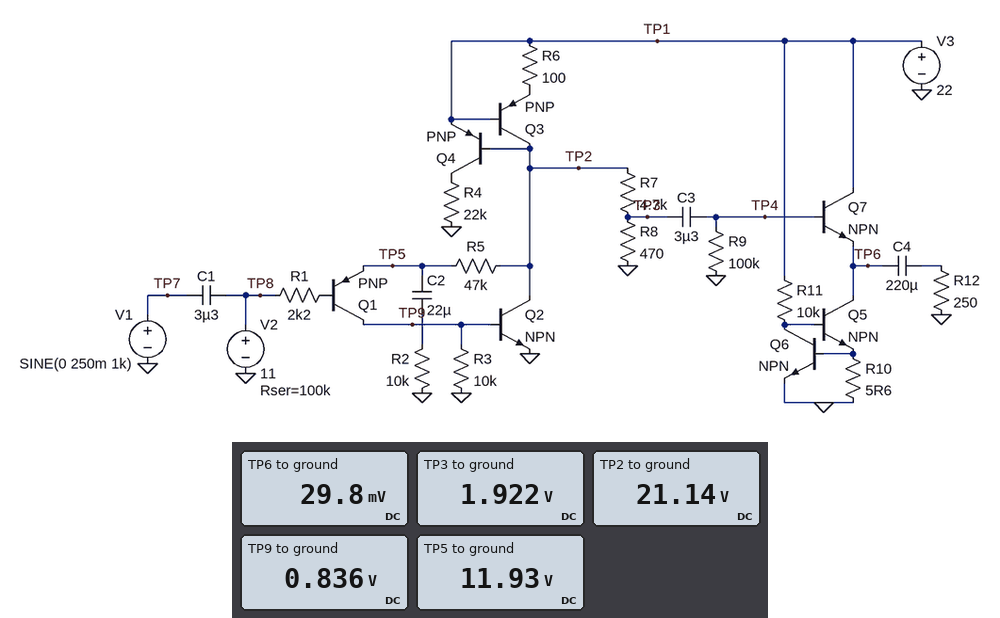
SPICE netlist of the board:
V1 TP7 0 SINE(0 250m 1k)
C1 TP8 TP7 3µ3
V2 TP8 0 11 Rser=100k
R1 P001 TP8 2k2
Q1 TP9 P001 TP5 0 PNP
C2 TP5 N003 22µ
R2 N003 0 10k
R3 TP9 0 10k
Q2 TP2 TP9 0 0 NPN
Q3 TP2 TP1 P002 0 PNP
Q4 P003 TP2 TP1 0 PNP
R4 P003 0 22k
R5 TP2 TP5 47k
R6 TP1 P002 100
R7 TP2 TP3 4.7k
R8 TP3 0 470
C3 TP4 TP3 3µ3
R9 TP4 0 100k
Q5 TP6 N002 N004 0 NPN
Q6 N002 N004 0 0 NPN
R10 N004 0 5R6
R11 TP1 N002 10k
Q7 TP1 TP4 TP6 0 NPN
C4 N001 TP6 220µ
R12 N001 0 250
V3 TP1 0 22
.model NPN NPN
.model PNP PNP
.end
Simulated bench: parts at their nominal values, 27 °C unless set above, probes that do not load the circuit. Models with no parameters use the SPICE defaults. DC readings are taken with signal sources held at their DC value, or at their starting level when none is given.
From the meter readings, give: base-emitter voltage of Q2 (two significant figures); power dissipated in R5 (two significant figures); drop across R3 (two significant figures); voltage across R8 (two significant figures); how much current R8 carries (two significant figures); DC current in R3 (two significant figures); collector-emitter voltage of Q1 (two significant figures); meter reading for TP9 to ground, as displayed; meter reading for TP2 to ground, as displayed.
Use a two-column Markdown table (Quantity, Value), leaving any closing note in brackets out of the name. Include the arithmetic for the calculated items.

| Quantity | Value |
|---|---|
| base-emitter voltage of Q2 | 836 mV = 840 mV |
| power dissipated in R5 | (21.14 V - 11.93 V)^2 / 47 kΩ = 1.8 mW |
| drop across R3 | 836 mV = 840 mV |
| voltage across R8 | 1.922 V = 1.9 V |
| how much current R8 carries | (1.922 V) / 470 Ω = 4.1 mA |
| DC current in R3 | (836 mV) / 10 kΩ = 84 µA |
| collector-emitter voltage of Q1 | 836 mV - 11.93 V = -11 V |
| meter reading for TP9 to ground, as displayed | 0.836 V |
| meter reading for TP2 to ground, as displayed | 21.14 V |
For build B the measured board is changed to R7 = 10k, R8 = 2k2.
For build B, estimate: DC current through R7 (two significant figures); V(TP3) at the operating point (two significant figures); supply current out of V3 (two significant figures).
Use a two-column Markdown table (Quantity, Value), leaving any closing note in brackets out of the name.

| Quantity | Value |
|---|---|
| DC current through R7 | 1.7 mA |
| V(TP3) at the operating point | 3.8 V |
| supply current out of V3 | 16 mA |
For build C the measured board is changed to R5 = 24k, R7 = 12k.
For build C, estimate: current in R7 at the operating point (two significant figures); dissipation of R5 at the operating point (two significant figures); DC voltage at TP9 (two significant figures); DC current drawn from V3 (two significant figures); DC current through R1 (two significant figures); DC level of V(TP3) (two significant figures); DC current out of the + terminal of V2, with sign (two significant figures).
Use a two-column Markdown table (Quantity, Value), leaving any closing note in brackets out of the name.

| Quantity | Value |
|---|---|
| current in R7 at the operating point | 1.7 mA |
| dissipation of R5 at the operating point | 3.4 mW |
| DC voltage at TP9 | 860 mV |
| DC current drawn from V3 | 34 mA |
| DC current through R1 | 3.7 µA |
| DC level of V(TP3) | 800 mV |
| DC current out of the + terminal of V2, with sign | -3.7 µA |
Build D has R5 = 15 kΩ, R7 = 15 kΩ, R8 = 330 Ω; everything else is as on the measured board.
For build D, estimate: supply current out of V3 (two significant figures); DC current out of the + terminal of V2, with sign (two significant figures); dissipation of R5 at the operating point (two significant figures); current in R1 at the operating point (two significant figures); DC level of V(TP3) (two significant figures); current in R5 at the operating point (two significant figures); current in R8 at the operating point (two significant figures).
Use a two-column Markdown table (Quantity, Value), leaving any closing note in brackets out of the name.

| Quantity | Value |
|---|---|
| supply current out of V3 | 54 mA |
| DC current out of the + terminal of V2, with sign | -5.8 µA |
| dissipation of R5 at the operating point | 5.1 mW |
| current in R1 at the operating point | 5.8 µA |
| DC level of V(TP3) | 450 mV |
| current in R5 at the operating point | 580 µA |
| current in R8 at the operating point | 1.4 mA |
